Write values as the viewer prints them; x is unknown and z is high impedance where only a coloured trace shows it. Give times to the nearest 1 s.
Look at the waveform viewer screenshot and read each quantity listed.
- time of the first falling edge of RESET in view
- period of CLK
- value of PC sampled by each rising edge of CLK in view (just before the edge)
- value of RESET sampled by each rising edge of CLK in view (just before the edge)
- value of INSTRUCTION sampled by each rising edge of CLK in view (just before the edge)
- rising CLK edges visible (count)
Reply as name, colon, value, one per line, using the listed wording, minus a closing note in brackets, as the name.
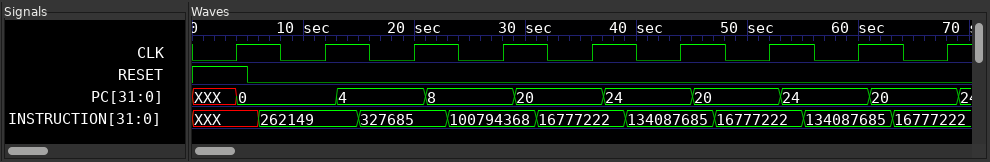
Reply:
time of the first falling edge of RESET in view: 5 s
period of CLK: 8 s
value of PC sampled by each rising edge of CLK in view: XXX, 0, 4, 8, 20, 24, 20, 24, 20
value of RESET sampled by each rising edge of CLK in view: 1 0 0 0 0 0 0 0 0
value of INSTRUCTION sampled by each rising edge of CLK in view: XXX, 262149, 327685, 100794368, 16777222, 134087685, 16777222, 134087685, 16777222
rising CLK edges visible: 9
